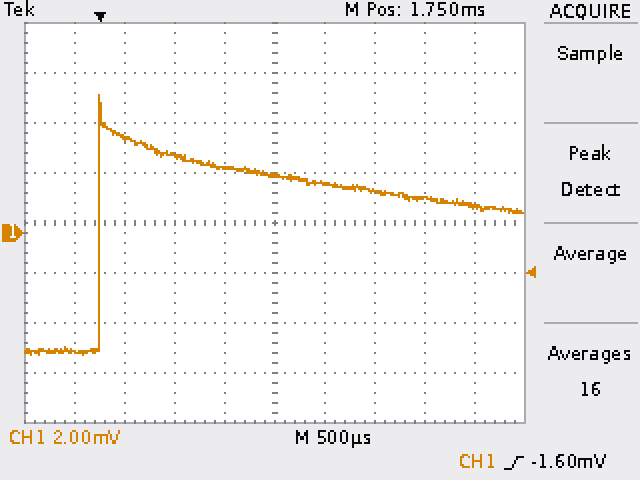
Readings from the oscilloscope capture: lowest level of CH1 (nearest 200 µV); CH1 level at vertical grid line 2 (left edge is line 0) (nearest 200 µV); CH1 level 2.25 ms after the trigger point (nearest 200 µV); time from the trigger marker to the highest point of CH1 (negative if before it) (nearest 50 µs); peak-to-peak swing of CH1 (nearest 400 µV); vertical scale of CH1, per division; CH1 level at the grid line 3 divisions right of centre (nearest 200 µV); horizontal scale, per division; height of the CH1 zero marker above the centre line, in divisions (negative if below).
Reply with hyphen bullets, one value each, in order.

- -4.8 mV
- 3.8 mV
- 2.0 mV
- 0 µs
- 10.4 mV
- 2 mV
- 1.4 mV
- 500 µs
- -0.2 div
